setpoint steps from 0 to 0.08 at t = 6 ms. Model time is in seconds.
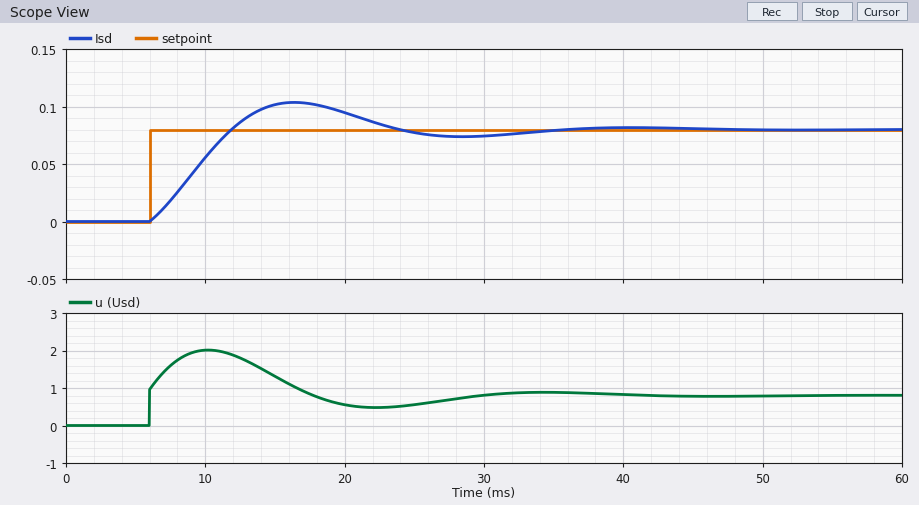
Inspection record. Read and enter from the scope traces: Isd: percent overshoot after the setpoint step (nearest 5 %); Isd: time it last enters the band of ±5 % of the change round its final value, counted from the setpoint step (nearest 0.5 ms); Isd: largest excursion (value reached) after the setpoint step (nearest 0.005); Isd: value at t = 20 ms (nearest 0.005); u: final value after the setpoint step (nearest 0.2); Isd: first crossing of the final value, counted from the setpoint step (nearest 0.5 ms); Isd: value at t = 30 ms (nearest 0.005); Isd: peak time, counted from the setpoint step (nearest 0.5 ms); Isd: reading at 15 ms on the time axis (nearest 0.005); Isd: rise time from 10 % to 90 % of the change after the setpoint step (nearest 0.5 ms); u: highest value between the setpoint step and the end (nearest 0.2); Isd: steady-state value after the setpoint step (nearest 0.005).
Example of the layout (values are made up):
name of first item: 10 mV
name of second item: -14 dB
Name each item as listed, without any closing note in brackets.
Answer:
Isd: percent overshoot after the setpoint step: 30 %
Isd: time it last enters the band of ±5 % of the change round its final value, counted from the setpoint step: 26.0 ms
Isd: largest excursion (value reached) after the setpoint step: 0.105
Isd: value at t = 20 ms: 0.095
u: final value after the setpoint step: 0.8
Isd: first crossing of the final value, counted from the setpoint step: 6.0 ms
Isd: value at t = 30 ms: 0.075
Isd: peak time, counted from the setpoint step: 10.5 ms
Isd: reading at 15 ms on the time axis: 0.100
Isd: rise time from 10 % to 90 % of the change after the setpoint step: 4.5 ms
u: highest value between the setpoint step and the end: 2.0
Isd: steady-state value after the setpoint step: 0.080
